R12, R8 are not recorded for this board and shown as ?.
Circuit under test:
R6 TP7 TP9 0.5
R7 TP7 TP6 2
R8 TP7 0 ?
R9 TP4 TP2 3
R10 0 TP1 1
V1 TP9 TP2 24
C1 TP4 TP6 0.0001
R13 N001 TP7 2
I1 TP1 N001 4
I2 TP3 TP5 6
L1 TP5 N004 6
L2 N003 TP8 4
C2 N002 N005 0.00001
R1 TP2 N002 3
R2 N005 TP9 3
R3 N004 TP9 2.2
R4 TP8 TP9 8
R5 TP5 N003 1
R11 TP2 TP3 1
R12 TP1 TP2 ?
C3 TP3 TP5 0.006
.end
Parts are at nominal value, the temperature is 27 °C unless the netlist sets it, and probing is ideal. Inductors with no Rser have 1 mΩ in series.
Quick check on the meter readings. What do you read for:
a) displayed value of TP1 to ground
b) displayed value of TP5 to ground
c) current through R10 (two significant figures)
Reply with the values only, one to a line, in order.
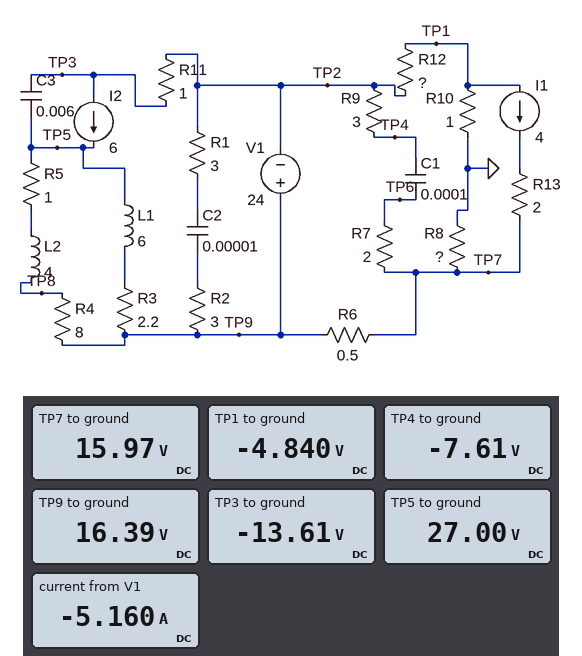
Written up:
-4.840 V
27.00 V
4.8 A
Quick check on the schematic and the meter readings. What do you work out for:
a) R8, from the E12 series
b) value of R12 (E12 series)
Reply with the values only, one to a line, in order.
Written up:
3.3 Ω
3.3 Ω
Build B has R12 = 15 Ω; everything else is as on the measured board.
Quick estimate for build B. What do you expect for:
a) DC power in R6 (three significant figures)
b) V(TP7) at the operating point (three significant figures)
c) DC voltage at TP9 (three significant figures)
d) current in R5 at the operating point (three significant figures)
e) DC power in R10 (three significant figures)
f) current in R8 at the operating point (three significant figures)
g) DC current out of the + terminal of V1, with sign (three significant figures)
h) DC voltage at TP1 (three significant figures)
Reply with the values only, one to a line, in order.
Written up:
59.0 mW
14.3 V
14.5 V
1.18 A
18.9 W
4.34 A
-5.66 A
-4.34 V
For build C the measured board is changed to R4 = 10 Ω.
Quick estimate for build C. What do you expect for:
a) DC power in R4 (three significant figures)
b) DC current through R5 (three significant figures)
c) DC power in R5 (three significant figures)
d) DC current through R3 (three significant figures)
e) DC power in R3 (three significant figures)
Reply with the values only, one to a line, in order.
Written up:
10.0 W
1.00 A
1.00 W
5.00 A
55.0 W
